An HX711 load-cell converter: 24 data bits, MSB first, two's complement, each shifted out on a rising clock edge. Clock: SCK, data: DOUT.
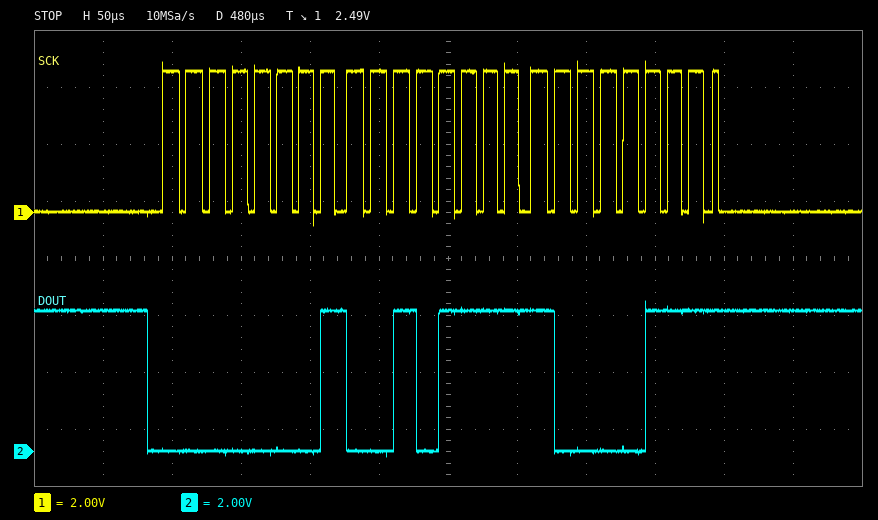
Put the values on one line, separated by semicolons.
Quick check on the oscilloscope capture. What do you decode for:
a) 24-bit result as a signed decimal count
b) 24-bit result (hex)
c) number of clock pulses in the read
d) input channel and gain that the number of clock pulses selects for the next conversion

77703; 0x012F87; 25; channel A, gain 128
